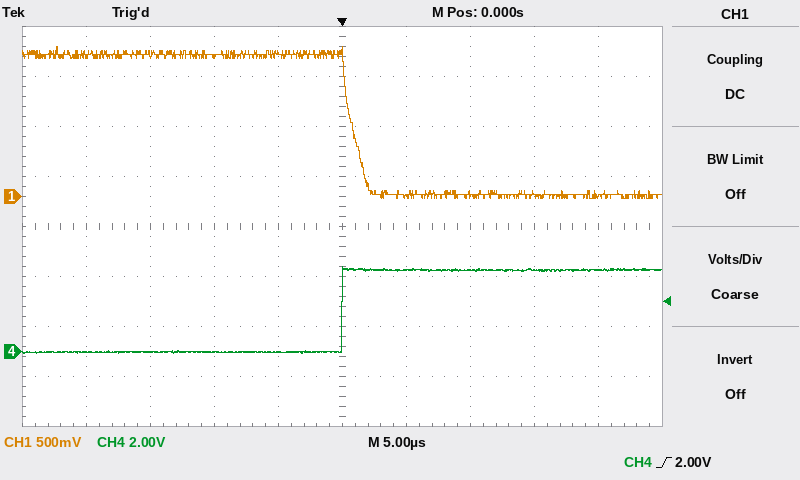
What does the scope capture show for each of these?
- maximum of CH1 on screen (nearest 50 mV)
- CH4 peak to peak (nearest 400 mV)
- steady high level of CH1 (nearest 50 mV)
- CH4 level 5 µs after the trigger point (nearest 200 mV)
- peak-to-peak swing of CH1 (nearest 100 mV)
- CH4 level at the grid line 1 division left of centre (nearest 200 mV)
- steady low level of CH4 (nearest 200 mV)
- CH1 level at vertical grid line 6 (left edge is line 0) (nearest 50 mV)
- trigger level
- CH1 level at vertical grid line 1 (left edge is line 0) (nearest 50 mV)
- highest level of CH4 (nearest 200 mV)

1.50 V
3.6 V
1.40 V
3.2 V
1.50 V
0.0 V
0.0 V
0 mV
2.00 V
1.40 V
3.4 V
